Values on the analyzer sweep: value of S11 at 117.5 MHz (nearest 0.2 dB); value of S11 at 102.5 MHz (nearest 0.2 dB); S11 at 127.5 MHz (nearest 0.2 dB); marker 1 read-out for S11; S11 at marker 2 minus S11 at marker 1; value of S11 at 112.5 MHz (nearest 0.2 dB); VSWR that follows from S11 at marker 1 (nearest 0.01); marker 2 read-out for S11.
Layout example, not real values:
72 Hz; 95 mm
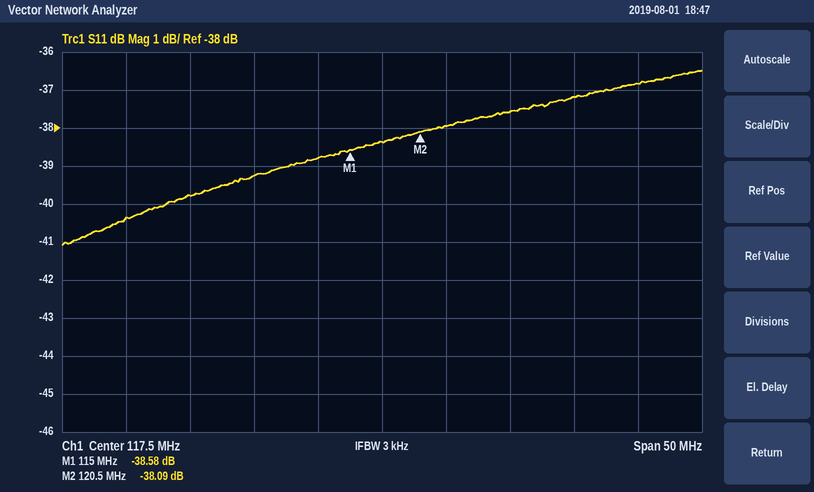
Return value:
-38.4 dB; -39.8 dB; -37.6 dB; -38.58 dB; 0.49 dB; -38.8 dB; 1.02; -38.09 dB
